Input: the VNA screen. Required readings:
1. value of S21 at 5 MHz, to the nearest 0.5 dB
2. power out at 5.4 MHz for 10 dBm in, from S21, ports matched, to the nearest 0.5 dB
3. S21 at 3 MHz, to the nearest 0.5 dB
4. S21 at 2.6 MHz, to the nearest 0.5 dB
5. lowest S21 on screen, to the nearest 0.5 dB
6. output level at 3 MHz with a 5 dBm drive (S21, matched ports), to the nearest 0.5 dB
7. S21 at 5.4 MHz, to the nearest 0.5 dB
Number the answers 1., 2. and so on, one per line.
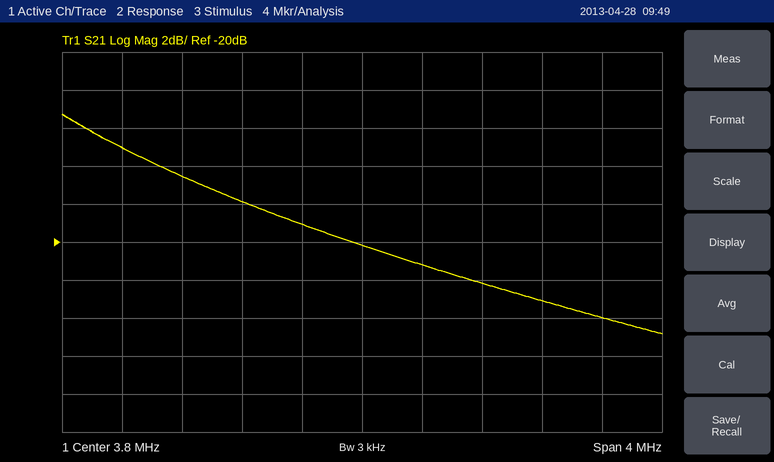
1. -23.0 dB
2. -14.0 dBm
3. -18.0 dB
4. -16.5 dB
5. -25.0 dB
6. -13.0 dBm
7. -24.0 dB
